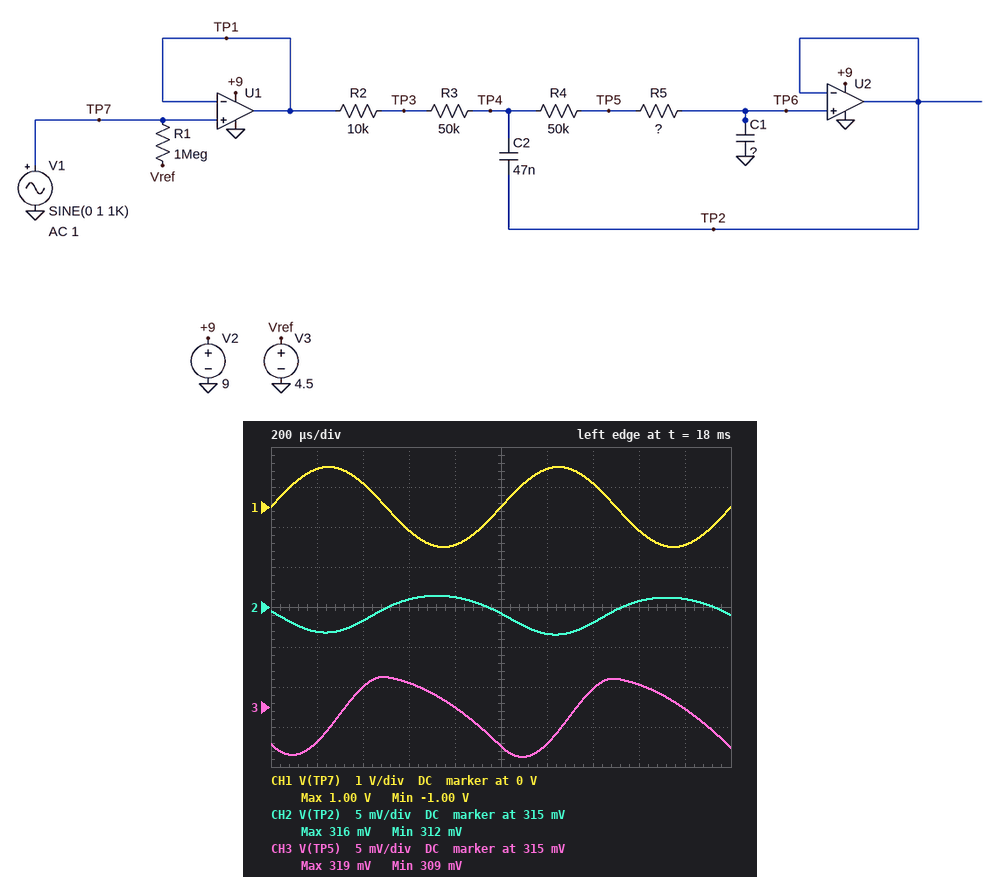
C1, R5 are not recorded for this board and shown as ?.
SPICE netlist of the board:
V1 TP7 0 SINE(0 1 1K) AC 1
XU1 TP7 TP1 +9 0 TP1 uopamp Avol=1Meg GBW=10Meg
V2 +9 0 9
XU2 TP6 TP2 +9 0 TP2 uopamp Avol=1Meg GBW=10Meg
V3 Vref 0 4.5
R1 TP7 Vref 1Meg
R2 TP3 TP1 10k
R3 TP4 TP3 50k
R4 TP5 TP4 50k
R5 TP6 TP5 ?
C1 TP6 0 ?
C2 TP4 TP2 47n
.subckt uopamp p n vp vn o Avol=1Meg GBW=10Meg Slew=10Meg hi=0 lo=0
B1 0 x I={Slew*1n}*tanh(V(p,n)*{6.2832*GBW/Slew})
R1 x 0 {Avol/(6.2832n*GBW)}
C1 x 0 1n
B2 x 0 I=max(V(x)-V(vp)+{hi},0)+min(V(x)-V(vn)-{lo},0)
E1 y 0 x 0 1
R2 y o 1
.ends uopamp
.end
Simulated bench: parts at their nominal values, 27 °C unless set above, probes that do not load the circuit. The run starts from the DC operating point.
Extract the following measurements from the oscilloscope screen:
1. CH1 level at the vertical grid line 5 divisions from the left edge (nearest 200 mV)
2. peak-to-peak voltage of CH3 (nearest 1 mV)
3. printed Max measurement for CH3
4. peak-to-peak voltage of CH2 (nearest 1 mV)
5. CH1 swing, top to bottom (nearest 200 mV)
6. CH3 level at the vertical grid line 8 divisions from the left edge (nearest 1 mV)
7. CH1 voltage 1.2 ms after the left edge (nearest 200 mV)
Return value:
0 V
10 mV
319 mV
5 mV
2.0 V
318 mV
1.0 V
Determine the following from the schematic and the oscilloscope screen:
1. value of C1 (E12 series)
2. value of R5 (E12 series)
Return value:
33 nF
8.2 kΩ
